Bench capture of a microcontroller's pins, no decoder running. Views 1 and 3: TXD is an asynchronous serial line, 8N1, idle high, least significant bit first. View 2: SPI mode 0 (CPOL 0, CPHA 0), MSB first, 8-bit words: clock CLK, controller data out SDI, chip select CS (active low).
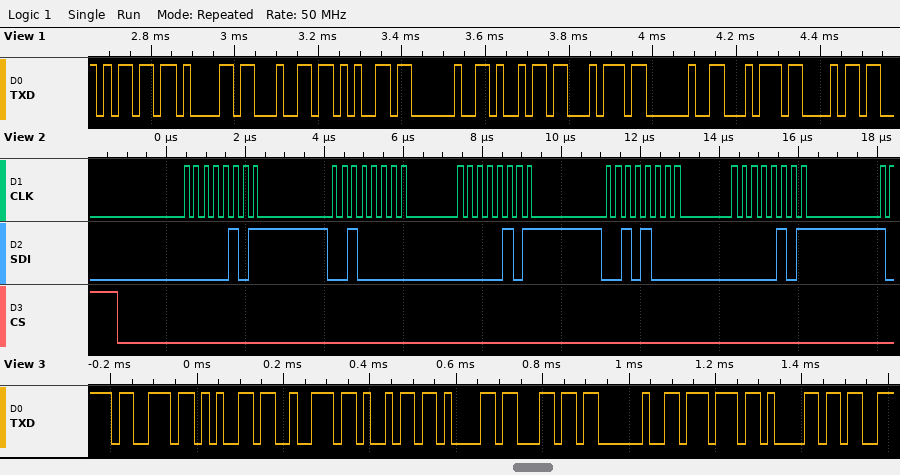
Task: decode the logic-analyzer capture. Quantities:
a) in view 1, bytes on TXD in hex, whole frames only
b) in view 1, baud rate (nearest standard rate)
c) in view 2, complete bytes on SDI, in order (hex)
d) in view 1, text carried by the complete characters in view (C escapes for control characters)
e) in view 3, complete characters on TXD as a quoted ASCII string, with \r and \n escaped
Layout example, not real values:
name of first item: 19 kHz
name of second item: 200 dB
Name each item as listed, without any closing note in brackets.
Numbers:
in view 1, bytes on TXD in hex, whole frames only: 6D 61 64 65 20 69 74 20 74 68
in view 1, baud rate: 57600 baud
in view 2, complete bytes on SDI, in order: 0x05 0x20 0x05 0x28 0x05
in view 1, text carried by the complete characters in view: "made it th"
in view 3, complete characters on TXD as a quoted ASCII string, with \r and \n escaped: "serial wa"
